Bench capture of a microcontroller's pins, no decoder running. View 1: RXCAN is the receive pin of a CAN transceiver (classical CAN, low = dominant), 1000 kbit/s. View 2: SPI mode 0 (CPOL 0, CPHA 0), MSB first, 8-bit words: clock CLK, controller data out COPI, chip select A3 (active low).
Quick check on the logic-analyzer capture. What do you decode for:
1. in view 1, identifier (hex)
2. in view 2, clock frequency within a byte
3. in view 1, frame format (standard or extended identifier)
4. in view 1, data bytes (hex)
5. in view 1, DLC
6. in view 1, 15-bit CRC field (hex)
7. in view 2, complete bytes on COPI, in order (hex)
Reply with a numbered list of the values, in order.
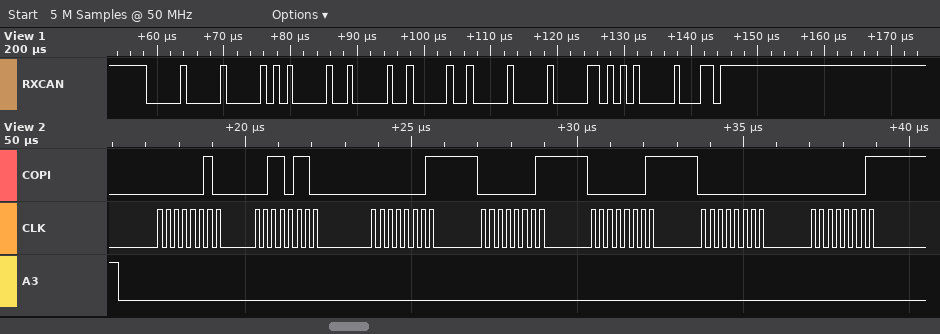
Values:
1. 0x000
2. 4 MHz
3. standard
4. 01 01 01 00 01
5. 5
6. 0x2A01
7. 02 36 01 01 01 00 01
